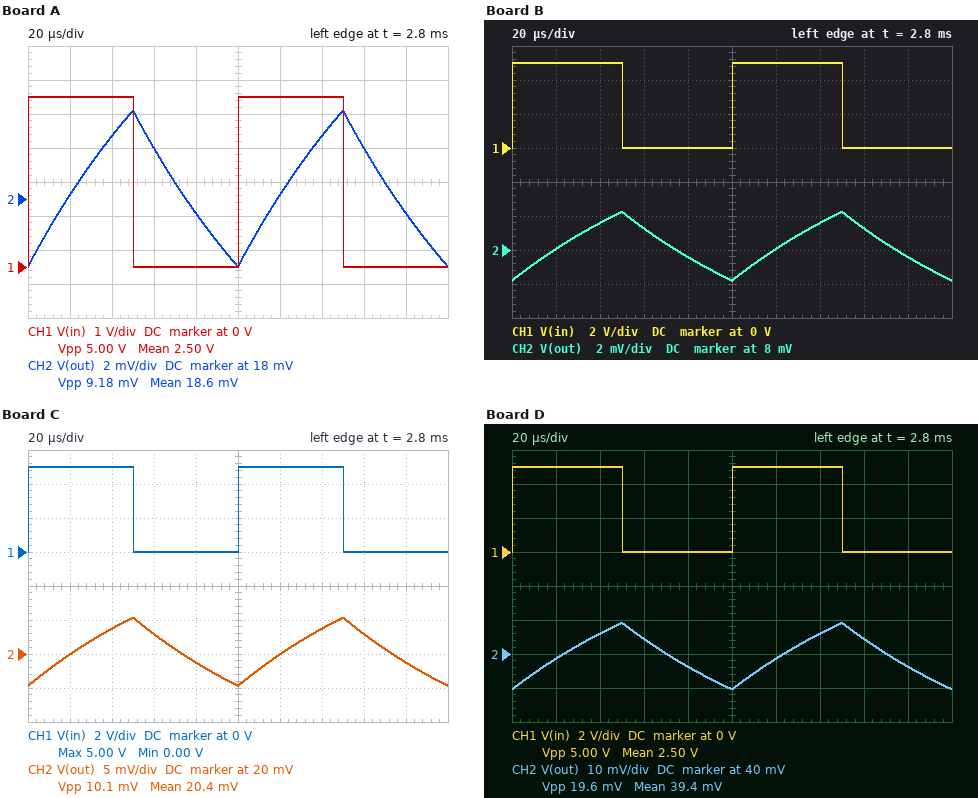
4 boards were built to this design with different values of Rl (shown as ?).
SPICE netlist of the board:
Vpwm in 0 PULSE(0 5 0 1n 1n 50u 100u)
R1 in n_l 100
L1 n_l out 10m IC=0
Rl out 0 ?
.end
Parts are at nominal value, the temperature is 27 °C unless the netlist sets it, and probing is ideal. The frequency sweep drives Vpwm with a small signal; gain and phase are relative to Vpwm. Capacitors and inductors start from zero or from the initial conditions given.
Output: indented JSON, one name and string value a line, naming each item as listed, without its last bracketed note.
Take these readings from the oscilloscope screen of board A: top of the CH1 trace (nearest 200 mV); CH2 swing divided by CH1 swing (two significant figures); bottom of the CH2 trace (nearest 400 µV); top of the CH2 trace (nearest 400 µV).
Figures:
{
  "top of the CH1 trace": "5.0 V",
  "CH2 swing divided by CH1 swing": "0.0018",
  "bottom of the CH2 trace": "14.0 mV",
  "top of the CH2 trace": "23.2 mV"
}
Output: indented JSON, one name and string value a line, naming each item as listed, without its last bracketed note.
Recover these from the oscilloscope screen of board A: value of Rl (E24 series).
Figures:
{
  "value of Rl": "0.75 Ω"
}
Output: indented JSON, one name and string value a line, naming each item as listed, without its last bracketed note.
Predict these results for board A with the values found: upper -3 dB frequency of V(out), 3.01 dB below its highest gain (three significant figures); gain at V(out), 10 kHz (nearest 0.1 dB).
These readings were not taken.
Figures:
{
  "upper -3 dB frequency of V(out), 3.01 dB below its highest gain": "1.60 kHz",
  "gain at V(out), 10 kHz": "-58.6 dB"
}
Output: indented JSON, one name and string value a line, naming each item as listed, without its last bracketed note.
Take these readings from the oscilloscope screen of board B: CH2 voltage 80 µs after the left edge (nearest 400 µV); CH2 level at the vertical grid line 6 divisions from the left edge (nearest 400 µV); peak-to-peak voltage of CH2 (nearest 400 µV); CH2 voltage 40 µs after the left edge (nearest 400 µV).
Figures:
{
  "CH2 voltage 80 µs after the left edge": "7.6 mV",
  "CH2 level at the vertical grid line 6 divisions from the left edge": "8.0 mV",
  "peak-to-peak voltage of CH2": "4.0 mV",
  "CH2 voltage 40 µs after the left edge": "9.6 mV"
}
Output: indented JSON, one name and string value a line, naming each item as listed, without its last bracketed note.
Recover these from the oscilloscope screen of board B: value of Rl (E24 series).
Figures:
{
  "value of Rl": "0.33 Ω"
}
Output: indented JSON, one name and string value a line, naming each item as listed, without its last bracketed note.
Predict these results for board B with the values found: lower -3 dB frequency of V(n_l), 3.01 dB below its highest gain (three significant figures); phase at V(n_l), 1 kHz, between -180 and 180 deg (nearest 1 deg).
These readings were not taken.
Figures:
{
  "lower -3 dB frequency of V(n_l), 3.01 dB below its highest gain": "1.60 kHz",
  "phase at V(n_l), 1 kHz, between -180 and 180 deg": "58 deg"
}
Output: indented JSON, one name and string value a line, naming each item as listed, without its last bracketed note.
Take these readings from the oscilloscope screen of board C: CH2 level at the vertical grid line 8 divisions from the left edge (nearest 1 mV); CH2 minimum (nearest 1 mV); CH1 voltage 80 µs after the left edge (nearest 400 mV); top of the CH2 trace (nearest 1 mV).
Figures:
{
  "CH2 level at the vertical grid line 8 divisions from the left edge": "23 mV",
  "CH2 minimum": "15 mV",
  "CH1 voltage 80 µs after the left edge": "0 V",
  "top of the CH2 trace": "25 mV"
}
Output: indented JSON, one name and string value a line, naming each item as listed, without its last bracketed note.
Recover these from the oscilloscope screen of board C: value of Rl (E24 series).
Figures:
{
  "value of Rl": "0.82 Ω"
}
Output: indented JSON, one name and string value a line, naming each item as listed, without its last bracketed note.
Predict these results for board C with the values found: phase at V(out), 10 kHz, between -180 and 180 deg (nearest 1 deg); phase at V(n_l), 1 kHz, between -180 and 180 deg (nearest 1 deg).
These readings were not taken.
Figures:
{
  "phase at V(out), 10 kHz, between -180 and 180 deg": "-81 deg",
  "phase at V(n_l), 1 kHz, between -180 and 180 deg": "57 deg"
}
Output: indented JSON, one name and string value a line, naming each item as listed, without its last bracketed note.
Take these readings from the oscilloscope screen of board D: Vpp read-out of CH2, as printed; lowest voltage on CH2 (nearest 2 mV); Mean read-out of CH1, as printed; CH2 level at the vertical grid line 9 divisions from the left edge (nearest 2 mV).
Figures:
{
  "Vpp read-out of CH2, as printed": "19.6 mV",
  "lowest voltage on CH2": "30 mV",
  "Mean read-out of CH1, as printed": "2.50 V",
  "CH2 level at the vertical grid line 9 divisions from the left edge": "36 mV"
}
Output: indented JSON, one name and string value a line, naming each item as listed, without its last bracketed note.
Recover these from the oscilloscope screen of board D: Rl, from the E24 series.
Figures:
{
  "Rl, from the E24 series": "1.6 Ω"
}
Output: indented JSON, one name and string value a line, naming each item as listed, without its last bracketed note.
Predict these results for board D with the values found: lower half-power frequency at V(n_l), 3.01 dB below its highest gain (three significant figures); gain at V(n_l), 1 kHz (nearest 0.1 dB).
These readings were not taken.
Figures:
{
  "lower half-power frequency at V(n_l), 3.01 dB below its highest gain": "1.62 kHz",
  "gain at V(n_l), 1 kHz": "-5.6 dB"
}
